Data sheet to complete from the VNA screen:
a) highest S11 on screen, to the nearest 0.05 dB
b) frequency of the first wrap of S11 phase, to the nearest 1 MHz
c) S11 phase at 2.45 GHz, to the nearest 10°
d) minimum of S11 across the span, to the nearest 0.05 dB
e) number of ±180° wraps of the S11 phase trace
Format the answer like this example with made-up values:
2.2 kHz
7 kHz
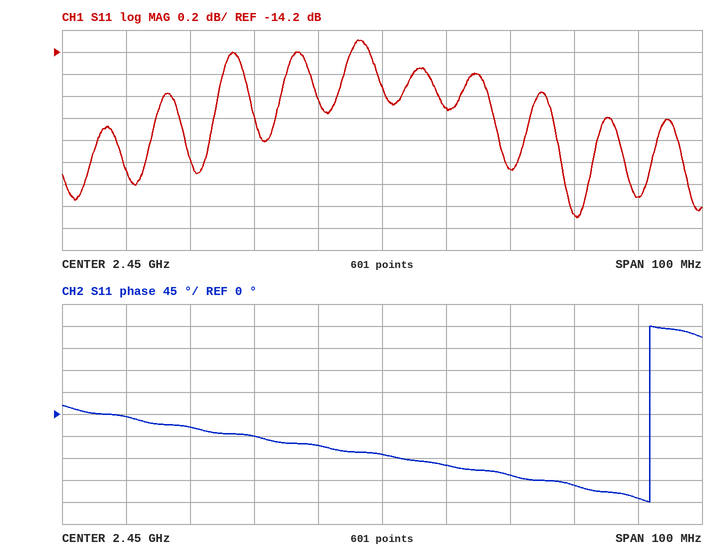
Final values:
-14.10 dB
2.492 GHz
-80°
-15.70 dB
1
